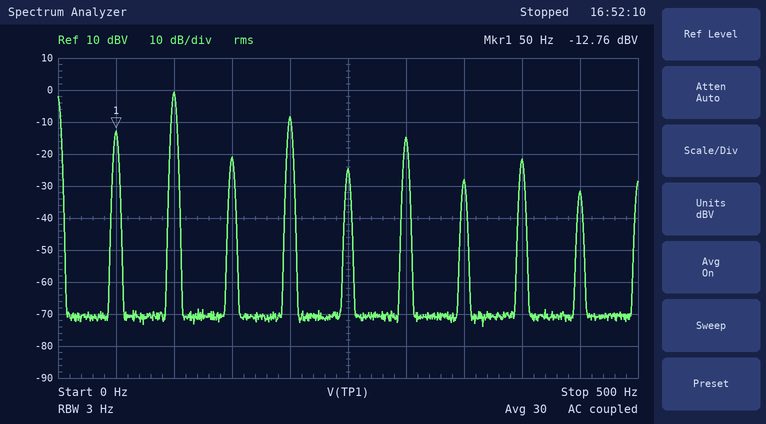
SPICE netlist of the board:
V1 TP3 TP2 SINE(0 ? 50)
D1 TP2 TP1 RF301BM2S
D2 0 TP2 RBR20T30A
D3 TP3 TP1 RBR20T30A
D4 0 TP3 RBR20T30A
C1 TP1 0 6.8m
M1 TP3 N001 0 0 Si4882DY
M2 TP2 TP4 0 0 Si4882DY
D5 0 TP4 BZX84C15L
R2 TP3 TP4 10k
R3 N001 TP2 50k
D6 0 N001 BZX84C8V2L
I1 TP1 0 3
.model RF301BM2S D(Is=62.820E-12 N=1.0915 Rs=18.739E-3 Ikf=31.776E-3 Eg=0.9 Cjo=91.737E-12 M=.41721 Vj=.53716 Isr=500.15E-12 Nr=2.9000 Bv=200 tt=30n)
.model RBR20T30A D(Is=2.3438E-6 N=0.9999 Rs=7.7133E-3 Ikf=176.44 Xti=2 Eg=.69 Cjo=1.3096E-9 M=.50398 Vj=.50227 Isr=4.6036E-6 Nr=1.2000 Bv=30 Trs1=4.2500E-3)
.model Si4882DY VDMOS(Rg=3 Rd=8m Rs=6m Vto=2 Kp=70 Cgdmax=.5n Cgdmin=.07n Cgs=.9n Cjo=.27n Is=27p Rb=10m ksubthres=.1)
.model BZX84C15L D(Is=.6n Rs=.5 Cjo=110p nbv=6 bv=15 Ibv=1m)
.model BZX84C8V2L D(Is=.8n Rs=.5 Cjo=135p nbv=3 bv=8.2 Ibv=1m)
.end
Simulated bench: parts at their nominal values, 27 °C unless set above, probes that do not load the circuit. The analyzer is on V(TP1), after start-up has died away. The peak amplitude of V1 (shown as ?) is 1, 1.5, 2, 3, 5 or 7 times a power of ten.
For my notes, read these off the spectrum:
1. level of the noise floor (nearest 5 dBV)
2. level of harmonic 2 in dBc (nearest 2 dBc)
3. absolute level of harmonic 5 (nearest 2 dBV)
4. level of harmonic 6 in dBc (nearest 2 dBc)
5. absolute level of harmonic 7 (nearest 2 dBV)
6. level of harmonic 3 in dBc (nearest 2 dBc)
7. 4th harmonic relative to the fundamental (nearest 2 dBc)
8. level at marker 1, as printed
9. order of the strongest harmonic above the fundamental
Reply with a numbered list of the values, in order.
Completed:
1. -70 dBV
2. 12 dBc
3. -24 dBV
4. -2 dBc
5. -28 dBV
6. -8 dBc
7. 4 dBc
8. -12.76 dBV
9. 2
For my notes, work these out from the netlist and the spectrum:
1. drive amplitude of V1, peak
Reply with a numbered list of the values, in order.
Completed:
1. 20 V
